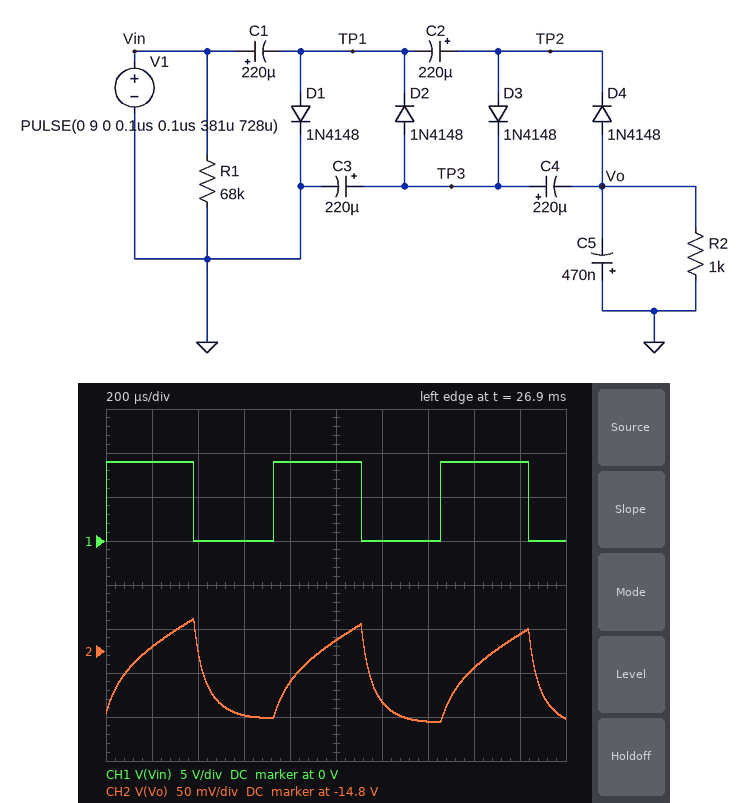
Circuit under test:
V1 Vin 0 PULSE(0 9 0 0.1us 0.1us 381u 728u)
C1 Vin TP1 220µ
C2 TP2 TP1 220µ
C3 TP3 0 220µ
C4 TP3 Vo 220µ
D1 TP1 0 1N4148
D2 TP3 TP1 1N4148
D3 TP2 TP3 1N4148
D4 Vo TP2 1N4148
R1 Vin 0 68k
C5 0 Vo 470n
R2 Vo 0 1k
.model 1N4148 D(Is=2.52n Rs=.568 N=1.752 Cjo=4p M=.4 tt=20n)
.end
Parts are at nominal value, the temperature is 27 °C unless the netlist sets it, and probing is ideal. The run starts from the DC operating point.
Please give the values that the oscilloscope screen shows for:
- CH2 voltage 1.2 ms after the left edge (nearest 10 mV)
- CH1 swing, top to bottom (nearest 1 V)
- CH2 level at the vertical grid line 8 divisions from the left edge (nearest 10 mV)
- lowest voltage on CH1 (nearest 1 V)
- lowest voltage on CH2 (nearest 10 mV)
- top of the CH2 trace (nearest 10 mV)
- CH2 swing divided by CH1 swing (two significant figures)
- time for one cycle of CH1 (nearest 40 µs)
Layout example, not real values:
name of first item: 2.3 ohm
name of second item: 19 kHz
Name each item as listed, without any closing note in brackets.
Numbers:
CH2 voltage 1.2 ms after the left edge: -14.86 V
CH1 swing, top to bottom: 9 V
CH2 level at the vertical grid line 8 divisions from the left edge: -14.82 V
lowest voltage on CH1: 0 V
lowest voltage on CH2: -14.88 V
top of the CH2 trace: -14.76 V
CH2 swing divided by CH1 swing: 0.013
time for one cycle of CH1: 720 µs
